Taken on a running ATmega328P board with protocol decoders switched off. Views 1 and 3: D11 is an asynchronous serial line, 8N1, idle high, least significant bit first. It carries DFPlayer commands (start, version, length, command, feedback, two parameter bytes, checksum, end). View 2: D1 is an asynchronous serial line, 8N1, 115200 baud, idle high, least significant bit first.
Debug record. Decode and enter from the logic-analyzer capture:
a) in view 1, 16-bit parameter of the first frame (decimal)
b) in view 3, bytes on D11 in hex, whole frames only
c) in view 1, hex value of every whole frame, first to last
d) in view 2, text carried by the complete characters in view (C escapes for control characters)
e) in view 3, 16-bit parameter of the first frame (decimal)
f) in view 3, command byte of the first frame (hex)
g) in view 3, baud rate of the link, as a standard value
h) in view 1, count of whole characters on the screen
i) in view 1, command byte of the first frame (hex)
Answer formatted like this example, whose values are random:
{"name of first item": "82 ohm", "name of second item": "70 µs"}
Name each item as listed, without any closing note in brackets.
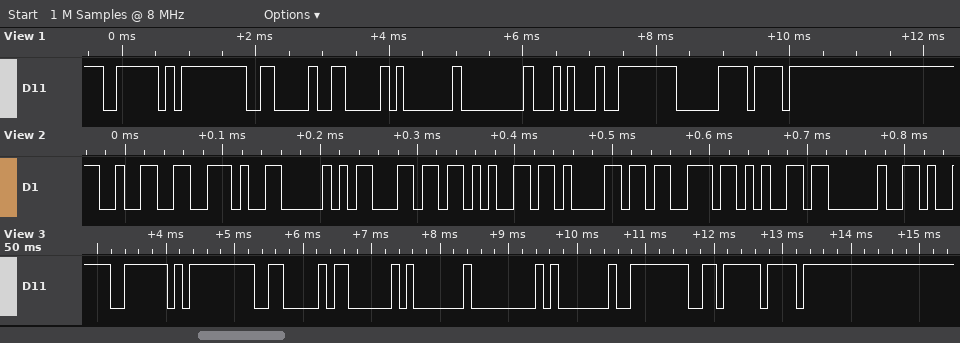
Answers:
{"in view 1, 16-bit parameter of the first frame": "20", "in view 3, bytes on D11 in hex, whole frames only": "0x7E 0xFF 0x06 0x03 0x01 0x00 0x01 0xFE 0xF6 0xEF", "in view 1, hex value of every whole frame, first to last": "7E FF 06 06 01 00 14 FE E0 EF", "in view 2, text carried by the complete characters in view": "\"2.Please \"", "in view 3, 16-bit parameter of the first frame": "1", "in view 3, command byte of the first frame": "0x03", "in view 3, baud rate of the link, as a standard value": "9600 baud", "in view 1, count of whole characters on the screen": "10", "in view 1, command byte of the first frame": "0x06"}
